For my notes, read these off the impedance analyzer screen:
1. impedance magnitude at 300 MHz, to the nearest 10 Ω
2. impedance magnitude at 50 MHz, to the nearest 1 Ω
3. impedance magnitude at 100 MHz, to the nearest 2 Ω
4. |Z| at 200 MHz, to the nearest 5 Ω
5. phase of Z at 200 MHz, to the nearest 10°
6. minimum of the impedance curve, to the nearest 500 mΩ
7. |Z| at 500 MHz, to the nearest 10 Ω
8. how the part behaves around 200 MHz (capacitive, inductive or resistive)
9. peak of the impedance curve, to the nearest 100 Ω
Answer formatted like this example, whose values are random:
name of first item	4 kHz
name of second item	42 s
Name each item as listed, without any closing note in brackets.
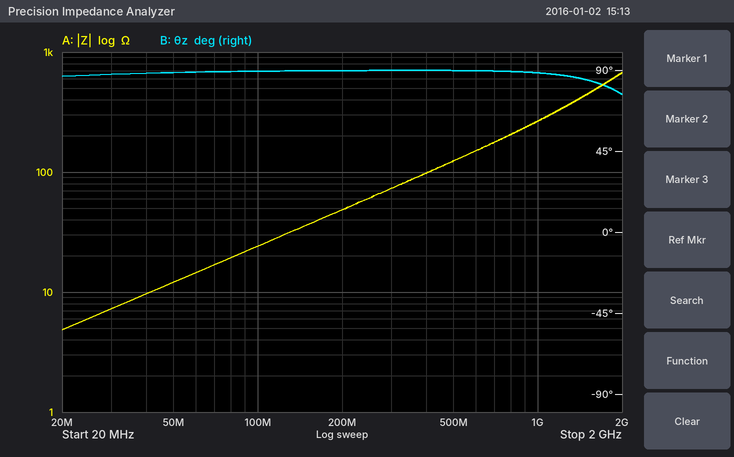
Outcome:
impedance magnitude at 300 MHz, to the nearest 10 Ω	70 Ω
impedance magnitude at 50 MHz, to the nearest 1 Ω	12 Ω
impedance magnitude at 100 MHz, to the nearest 2 Ω	24 Ω
|Z| at 200 MHz, to the nearest 5 Ω	50 Ω
phase of Z at 200 MHz, to the nearest 10°	90°
minimum of the impedance curve, to the nearest 500 mΩ	5.0 Ω
|Z| at 500 MHz, to the nearest 10 Ω	120 Ω
how the part behaves around 200 MHz	inductive
peak of the impedance curve, to the nearest 100 Ω	700 Ω
